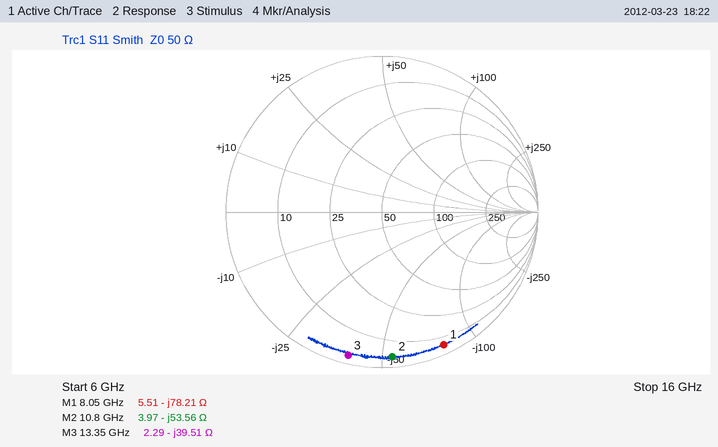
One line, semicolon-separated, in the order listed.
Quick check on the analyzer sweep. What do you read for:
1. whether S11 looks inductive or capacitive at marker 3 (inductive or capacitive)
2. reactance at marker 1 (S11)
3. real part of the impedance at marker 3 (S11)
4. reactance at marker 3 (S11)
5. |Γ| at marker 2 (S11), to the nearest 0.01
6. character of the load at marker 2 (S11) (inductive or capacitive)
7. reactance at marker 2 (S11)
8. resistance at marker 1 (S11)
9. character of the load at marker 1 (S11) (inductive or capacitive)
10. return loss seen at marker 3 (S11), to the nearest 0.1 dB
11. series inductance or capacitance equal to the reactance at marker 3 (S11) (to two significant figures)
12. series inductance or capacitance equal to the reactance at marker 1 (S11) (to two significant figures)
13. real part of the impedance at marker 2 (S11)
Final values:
capacitive; -78.21 Ω; 2.29 Ω; -39.51 Ω; 0.93; capacitive; -53.56 Ω; 5.51 Ω; capacitive; 0.5 dB; 300 fF; 250 fF; 3.97 Ω
